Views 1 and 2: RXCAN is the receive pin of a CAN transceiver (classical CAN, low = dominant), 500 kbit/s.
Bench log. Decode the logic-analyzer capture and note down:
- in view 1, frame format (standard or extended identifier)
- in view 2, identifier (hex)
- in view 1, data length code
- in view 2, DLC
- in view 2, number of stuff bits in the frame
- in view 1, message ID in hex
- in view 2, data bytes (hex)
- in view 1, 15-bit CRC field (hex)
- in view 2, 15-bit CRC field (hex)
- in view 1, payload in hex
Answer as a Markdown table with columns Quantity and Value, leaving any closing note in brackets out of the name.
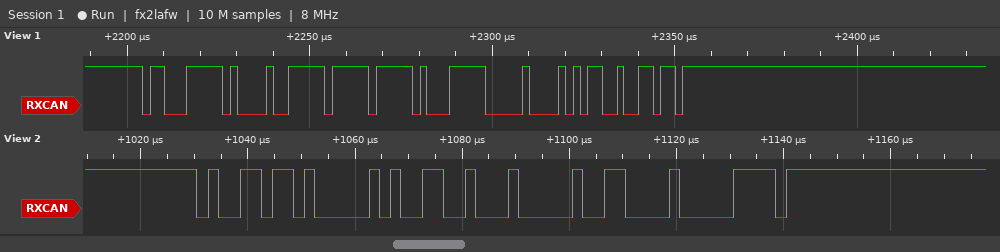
| Quantity | Value |
|---|---|
| in view 1, frame format | standard |
| in view 2, identifier | 0x4DA |
| in view 1, data length code | 4 |
| in view 2, DLC | 2 |
| in view 2, number of stuff bits in the frame | 3 |
| in view 1, message ID in hex | 0x63F |
| in view 2, data bytes | 64 40 |
| in view 1, 15-bit CRC field | 0x564D |
| in view 2, 15-bit CRC field | 0x3083 |
| in view 1, payload in hex | FF FF 1F 00 |
